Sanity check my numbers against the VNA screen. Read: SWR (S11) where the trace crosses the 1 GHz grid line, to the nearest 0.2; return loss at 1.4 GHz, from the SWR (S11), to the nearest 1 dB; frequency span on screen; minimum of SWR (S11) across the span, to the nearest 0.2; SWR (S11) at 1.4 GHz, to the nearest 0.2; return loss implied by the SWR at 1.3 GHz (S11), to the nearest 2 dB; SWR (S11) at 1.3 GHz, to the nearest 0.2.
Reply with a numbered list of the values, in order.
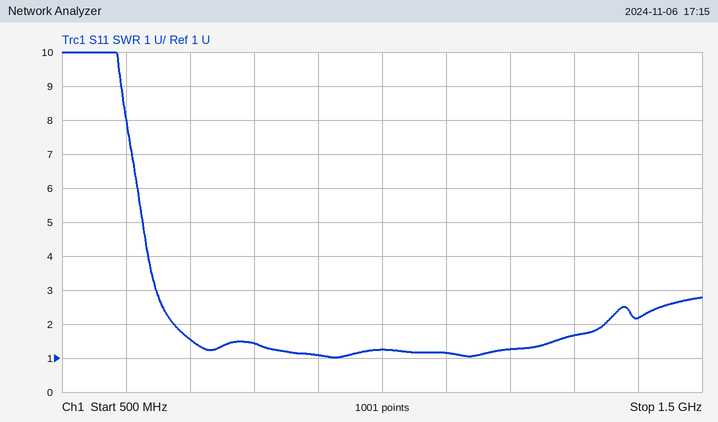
1. 1.2
2. 9 dB
3. 1 GHz
4. 1.0
5. 2.2
6. 12 dB
7. 1.6
